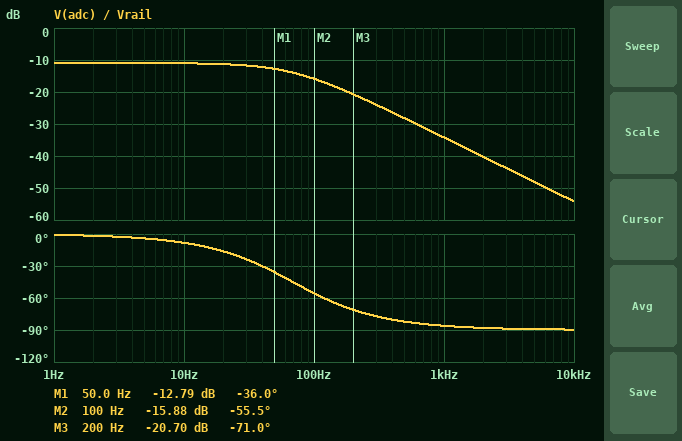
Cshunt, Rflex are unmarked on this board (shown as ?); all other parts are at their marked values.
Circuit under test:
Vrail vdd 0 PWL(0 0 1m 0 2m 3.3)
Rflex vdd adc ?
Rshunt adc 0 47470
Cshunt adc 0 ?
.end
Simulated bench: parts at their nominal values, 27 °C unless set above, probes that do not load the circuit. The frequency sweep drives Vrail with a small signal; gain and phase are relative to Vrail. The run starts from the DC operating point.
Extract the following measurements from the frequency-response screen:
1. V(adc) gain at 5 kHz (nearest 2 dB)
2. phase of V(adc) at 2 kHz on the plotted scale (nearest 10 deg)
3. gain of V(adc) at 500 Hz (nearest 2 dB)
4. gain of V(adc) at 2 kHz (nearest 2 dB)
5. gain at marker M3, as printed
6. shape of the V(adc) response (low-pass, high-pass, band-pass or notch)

-48 dB
-90 deg
-28 dB
-40 dB
-20.70 dB
low-pass
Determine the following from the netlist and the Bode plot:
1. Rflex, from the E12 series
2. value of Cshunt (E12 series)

120 kΩ
68 nF
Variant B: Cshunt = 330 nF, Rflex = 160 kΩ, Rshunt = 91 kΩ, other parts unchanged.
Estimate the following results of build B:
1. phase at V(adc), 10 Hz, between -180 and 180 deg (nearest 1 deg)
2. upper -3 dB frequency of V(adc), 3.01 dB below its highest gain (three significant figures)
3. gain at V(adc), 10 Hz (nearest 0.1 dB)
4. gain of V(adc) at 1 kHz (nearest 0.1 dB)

-50 deg
8.31 Hz
-12.7 dB
-50.4 dB
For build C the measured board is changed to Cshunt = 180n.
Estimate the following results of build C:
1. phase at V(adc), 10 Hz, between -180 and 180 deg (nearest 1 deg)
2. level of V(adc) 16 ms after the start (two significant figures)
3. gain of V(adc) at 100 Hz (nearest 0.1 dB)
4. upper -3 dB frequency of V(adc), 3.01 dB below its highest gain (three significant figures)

-21 deg
850 mV
-22.9 dB
26.0 Hz
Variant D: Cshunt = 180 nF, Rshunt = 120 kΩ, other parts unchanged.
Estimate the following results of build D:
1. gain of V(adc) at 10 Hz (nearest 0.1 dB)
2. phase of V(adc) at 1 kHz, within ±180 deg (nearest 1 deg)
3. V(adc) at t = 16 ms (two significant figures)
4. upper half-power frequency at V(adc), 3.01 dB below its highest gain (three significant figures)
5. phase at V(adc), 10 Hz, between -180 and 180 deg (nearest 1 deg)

-7.7 dB
-89 deg
1.2 V
14.7 Hz
-34 deg
